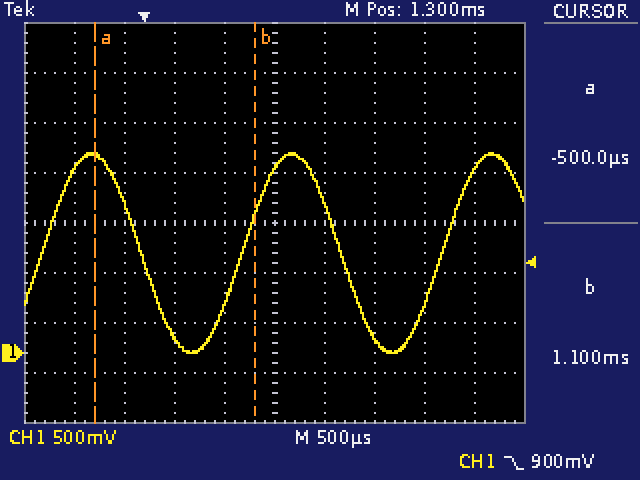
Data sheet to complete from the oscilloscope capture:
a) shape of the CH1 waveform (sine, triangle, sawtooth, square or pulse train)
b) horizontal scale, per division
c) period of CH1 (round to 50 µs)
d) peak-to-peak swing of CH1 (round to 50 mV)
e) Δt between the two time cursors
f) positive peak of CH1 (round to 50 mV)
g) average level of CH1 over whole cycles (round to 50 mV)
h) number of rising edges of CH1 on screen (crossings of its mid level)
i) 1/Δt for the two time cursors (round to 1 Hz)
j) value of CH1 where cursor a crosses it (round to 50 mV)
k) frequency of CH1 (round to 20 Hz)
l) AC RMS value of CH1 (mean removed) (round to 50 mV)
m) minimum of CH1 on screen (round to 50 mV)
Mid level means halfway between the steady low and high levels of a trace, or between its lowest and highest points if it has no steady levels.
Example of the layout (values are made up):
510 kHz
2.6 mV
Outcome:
sine
500 µs
2.00 ms
2.00 V
1.60 ms
2.00 V
1.00 V
3
625 Hz
1.95 V
500 Hz
700 mV
0 mV
